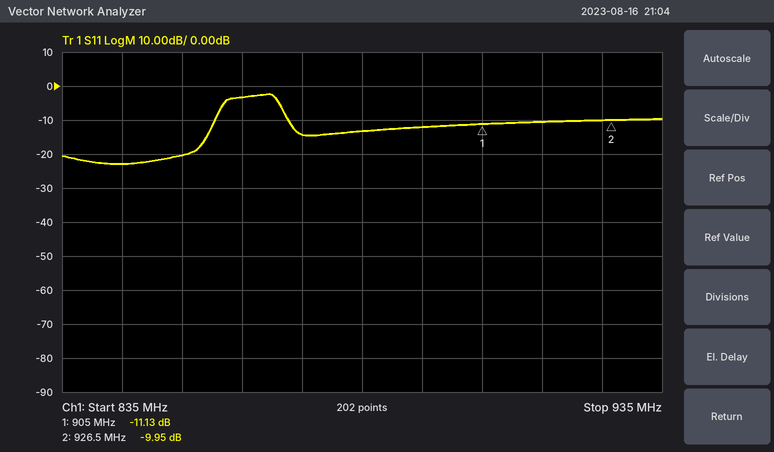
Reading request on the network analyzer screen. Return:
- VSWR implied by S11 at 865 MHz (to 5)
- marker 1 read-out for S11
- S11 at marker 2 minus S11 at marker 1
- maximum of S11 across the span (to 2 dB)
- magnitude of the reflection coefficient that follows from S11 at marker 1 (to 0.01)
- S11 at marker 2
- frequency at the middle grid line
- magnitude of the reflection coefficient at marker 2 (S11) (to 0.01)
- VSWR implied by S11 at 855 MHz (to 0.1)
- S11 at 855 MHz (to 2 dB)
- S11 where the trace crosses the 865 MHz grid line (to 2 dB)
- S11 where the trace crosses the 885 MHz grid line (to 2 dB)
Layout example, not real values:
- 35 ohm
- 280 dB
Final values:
- 5
- -11.13 dB
- 1.18 dB
- -2 dB
- 0.28
- -9.95 dB
- 885 MHz
- 0.32
- 1.2
- -20 dB
- -4 dB
- -14 dB
